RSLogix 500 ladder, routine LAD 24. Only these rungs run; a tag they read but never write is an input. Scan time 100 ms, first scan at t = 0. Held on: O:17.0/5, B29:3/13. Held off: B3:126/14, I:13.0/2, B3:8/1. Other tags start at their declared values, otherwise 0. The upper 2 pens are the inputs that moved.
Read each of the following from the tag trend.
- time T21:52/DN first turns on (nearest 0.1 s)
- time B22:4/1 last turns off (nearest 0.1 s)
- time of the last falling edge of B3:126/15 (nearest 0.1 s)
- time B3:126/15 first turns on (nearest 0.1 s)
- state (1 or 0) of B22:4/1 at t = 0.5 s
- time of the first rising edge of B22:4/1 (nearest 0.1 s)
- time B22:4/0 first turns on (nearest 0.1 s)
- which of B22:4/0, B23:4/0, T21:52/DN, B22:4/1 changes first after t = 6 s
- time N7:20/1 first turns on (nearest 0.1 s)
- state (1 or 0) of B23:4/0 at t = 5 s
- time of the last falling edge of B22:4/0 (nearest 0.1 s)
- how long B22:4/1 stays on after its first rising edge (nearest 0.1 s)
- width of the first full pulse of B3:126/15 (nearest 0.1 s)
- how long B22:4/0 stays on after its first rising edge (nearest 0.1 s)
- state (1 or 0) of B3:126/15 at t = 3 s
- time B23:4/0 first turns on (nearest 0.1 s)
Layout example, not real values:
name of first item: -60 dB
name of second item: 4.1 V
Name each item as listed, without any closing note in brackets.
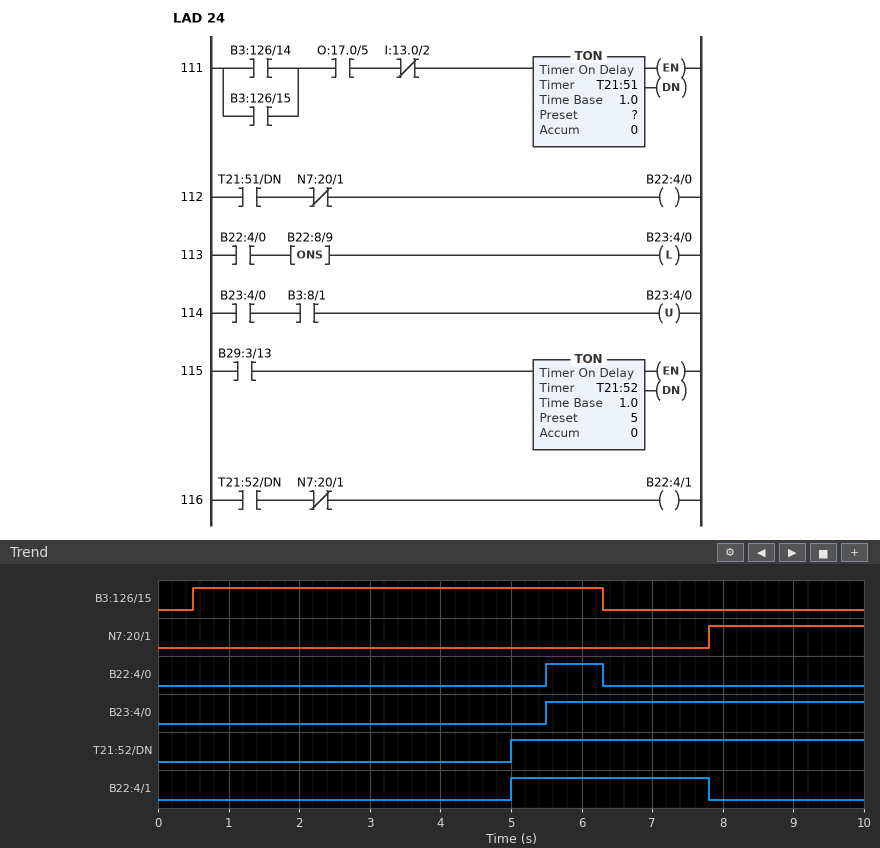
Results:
time T21:52/DN first turns on: 5.0 s
time B22:4/1 last turns off: 7.8 s
time of the last falling edge of B3:126/15: 6.3 s
time B3:126/15 first turns on: 0.5 s
state (1 or 0) of B22:4/1 at t = 0.5 s: 0
time of the first rising edge of B22:4/1: 5.0 s
time B22:4/0 first turns on: 5.5 s
which of B22:4/0, B23:4/0, T21:52/DN, B22:4/1 changes first after t = 6 s: B22:4/0
time N7:20/1 first turns on: 7.8 s
state (1 or 0) of B23:4/0 at t = 5 s: 0
time of the last falling edge of B22:4/0: 6.3 s
how long B22:4/1 stays on after its first rising edge: 2.8 s
width of the first full pulse of B3:126/15: 5.8 s
how long B22:4/0 stays on after its first rising edge: 0.8 s
state (1 or 0) of B3:126/15 at t = 3 s: 1
time B23:4/0 first turns on: 5.5 s
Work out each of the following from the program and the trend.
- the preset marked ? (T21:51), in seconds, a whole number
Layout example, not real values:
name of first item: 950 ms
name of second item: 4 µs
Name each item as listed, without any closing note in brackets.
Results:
the preset marked ? (T21:51), in seconds, a whole number: 5 s
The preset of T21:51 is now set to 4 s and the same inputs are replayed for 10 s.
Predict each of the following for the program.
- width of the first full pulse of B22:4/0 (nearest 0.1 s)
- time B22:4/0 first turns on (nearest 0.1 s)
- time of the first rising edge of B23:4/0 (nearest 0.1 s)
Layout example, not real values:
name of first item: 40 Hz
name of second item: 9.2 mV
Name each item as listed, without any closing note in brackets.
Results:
width of the first full pulse of B22:4/0: 1.8 s
time B22:4/0 first turns on: 4.5 s
time of the first rising edge of B23:4/0: 4.5 s
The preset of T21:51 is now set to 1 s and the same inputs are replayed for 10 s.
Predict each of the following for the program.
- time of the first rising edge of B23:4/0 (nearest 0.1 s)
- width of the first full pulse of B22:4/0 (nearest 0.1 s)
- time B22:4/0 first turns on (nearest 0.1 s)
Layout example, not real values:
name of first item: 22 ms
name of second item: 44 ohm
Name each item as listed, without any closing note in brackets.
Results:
time of the first rising edge of B23:4/0: 1.5 s
width of the first full pulse of B22:4/0: 4.8 s
time B22:4/0 first turns on: 1.5 s
